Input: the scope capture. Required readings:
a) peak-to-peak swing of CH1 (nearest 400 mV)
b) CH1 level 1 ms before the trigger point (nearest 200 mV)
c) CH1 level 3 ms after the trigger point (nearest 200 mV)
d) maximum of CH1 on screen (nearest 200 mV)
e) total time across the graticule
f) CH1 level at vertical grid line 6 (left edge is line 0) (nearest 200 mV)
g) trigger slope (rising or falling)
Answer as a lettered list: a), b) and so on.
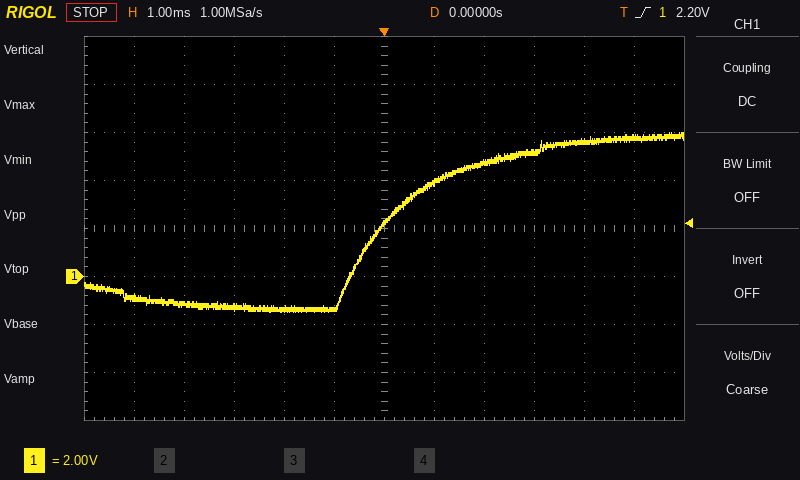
a) 7.6 V
b) -1.4 V
c) 5.2 V
d) 6.0 V
e) 12 ms
f) 2.2 V
g) rising
